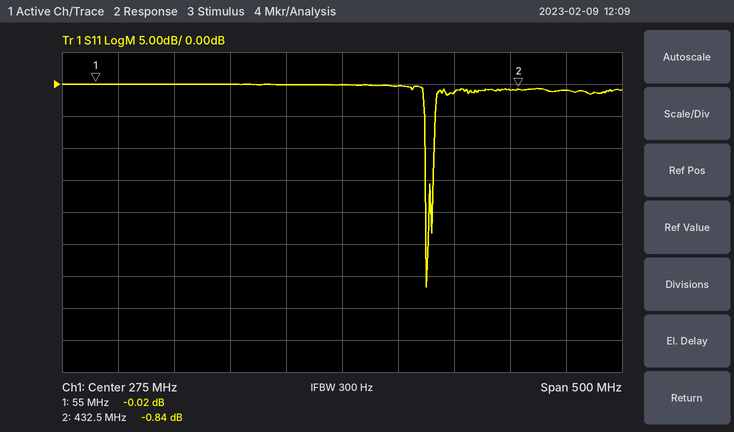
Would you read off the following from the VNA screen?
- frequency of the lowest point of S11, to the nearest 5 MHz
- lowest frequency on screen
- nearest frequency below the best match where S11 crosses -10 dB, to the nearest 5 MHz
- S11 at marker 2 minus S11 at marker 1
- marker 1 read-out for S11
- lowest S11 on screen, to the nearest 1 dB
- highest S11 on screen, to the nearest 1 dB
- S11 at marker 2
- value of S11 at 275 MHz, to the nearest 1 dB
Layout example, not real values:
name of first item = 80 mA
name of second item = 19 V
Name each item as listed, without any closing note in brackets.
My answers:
frequency of the lowest point of S11, to the nearest 5 MHz = 350 MHz
lowest frequency on screen = 25 MHz
nearest frequency below the best match where S11 crosses -10 dB, to the nearest 5 MHz = 350 MHz
S11 at marker 2 minus S11 at marker 1 = -0.82 dB
marker 1 read-out for S11 = -0.02 dB
lowest S11 on screen, to the nearest 1 dB = -32 dB
highest S11 on screen, to the nearest 1 dB = 0 dB
S11 at marker 2 = -0.84 dB
value of S11 at 275 MHz, to the nearest 1 dB = 0 dB
